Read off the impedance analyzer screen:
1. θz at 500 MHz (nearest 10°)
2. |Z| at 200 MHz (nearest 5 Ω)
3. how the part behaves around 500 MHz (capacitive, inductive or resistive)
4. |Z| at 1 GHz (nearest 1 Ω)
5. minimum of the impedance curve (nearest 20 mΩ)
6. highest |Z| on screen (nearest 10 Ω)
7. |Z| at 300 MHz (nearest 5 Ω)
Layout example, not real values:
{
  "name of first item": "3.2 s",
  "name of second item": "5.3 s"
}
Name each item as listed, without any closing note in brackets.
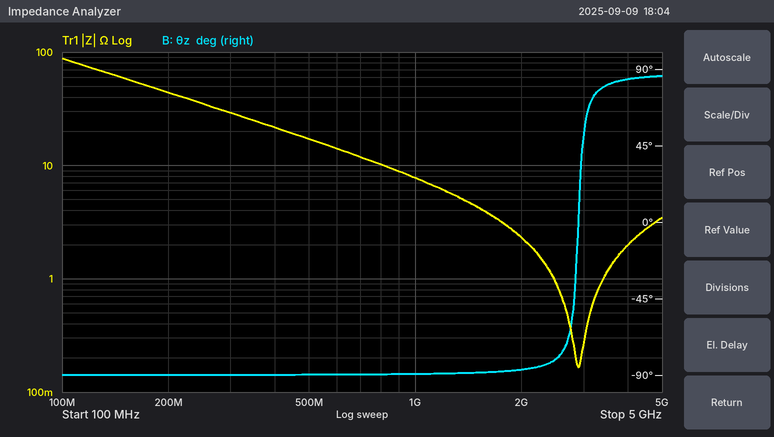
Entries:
{
  "θz at 500 MHz": "-90°",
  "|Z| at 200 MHz": "45 Ω",
  "how the part behaves around 500 MHz": "capacitive",
  "|Z| at 1 GHz": "8 Ω",
  "minimum of the impedance curve": "160 mΩ",
  "highest |Z| on screen": "90 Ω",
  "|Z| at 300 MHz": "30 Ω"
}
